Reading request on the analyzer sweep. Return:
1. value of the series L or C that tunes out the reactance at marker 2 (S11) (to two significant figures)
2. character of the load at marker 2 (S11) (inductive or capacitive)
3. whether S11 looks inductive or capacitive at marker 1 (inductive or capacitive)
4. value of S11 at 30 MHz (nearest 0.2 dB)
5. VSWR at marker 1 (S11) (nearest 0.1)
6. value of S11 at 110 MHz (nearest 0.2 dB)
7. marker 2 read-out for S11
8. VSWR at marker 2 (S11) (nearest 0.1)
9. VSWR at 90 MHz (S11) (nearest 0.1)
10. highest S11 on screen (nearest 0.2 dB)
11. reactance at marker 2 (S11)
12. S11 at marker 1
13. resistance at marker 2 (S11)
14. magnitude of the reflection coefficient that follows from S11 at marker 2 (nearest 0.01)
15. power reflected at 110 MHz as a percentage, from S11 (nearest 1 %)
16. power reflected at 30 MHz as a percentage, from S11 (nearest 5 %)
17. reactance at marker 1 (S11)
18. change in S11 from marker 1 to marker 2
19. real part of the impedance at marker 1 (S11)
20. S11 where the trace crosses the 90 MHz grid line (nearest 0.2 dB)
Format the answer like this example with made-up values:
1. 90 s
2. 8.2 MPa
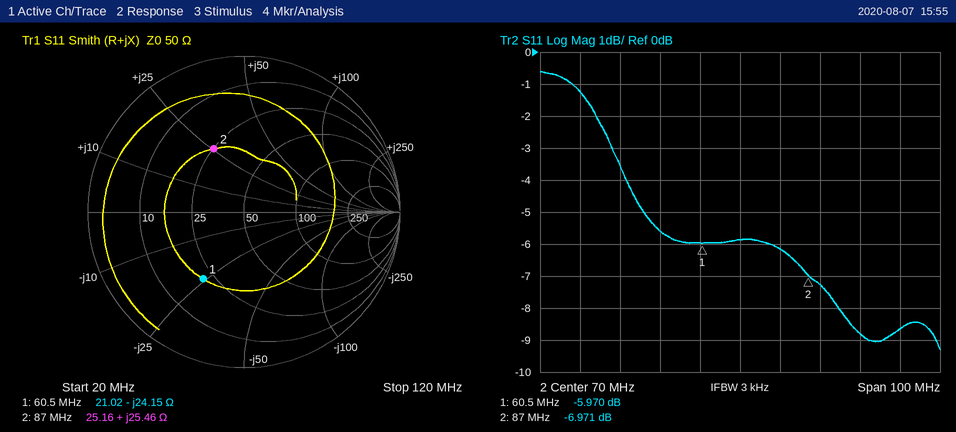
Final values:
1. 72 pF
2. inductive
3. capacitive
4. -1.2 dB
5. 3.0
6. -8.6 dB
7. -6.971 dB
8. 2.6
9. 2.5
10. -0.6 dB
11. +25.46 Ω
12. -5.970 dB
13. 25.16 Ω
14. 0.45
15. 14 %
16. 75 %
17. -24.15 Ω
18. -1.001 dB
19. 21.02 Ω
20. -7.2 dB
